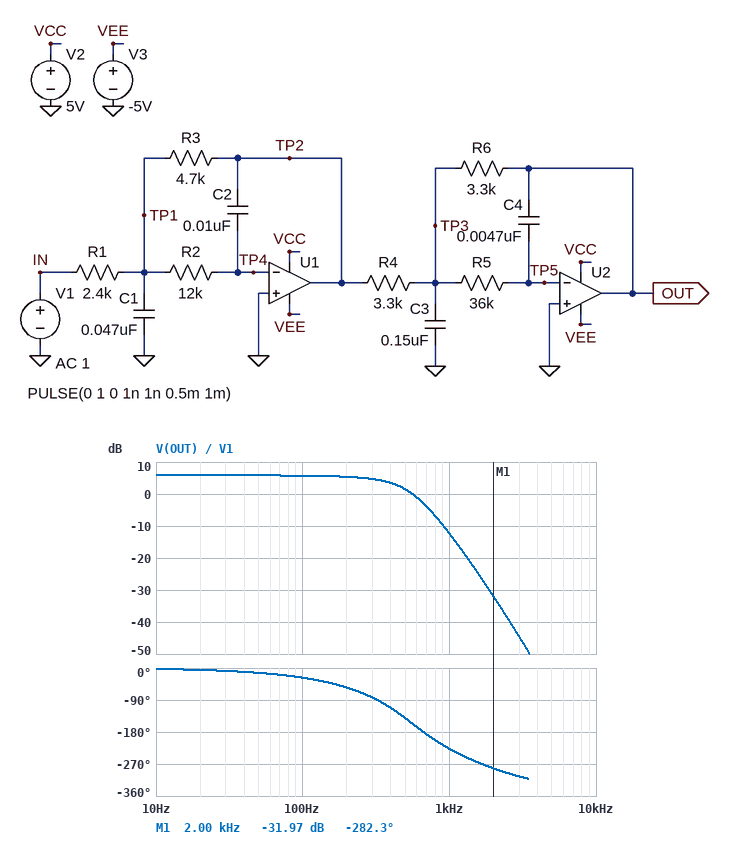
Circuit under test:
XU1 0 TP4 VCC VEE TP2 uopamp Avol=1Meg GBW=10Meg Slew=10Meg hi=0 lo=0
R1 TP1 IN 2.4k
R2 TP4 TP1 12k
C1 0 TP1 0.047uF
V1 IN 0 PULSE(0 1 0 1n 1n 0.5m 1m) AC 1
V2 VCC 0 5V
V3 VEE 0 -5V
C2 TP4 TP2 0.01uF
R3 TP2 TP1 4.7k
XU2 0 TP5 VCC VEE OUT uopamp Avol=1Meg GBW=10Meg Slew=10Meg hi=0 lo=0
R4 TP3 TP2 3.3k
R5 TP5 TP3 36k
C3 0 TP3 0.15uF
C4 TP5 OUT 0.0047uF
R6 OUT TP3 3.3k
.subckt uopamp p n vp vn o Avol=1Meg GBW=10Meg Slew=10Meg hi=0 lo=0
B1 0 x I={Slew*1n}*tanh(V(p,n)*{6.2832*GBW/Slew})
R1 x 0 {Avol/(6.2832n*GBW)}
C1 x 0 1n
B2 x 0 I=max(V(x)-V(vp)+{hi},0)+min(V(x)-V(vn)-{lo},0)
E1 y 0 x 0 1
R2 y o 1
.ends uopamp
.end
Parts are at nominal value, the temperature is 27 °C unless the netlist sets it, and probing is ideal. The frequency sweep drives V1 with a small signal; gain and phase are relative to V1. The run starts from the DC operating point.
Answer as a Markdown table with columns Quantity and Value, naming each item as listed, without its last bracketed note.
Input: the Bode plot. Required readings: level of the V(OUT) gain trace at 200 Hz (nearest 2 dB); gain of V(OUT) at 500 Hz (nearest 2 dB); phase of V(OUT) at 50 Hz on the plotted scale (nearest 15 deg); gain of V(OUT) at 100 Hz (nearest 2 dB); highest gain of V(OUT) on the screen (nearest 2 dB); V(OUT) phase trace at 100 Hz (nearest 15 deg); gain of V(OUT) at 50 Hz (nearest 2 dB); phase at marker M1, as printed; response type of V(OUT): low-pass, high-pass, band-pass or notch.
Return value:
| Quantity | Value |
|---|---|
| level of the V(OUT) gain trace at 200 Hz | 6 dB |
| gain of V(OUT) at 500 Hz | 2 dB |
| phase of V(OUT) at 50 Hz on the plotted scale | -15 deg |
| gain of V(OUT) at 100 Hz | 6 dB |
| highest gain of V(OUT) on the screen | 6 dB |
| V(OUT) phase trace at 100 Hz | -30 deg |
| gain of V(OUT) at 50 Hz | 6 dB |
| phase at marker M1, as printed | -282.3 deg |
| response type of V(OUT): low-pass, high-pass, band-pass or notch | low-pass |
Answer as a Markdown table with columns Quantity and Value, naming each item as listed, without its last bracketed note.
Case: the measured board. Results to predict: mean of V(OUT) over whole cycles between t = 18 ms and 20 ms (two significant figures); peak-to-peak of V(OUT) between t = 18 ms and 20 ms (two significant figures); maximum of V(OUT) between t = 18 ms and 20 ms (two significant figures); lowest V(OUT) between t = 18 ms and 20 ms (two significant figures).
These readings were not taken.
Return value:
| Quantity | Value |
|---|---|
| mean of V(OUT) over whole cycles between t = 18 ms and 20 ms | 980 mV |
| peak-to-peak of V(OUT) between t = 18 ms and 20 ms | 310 mV |
| maximum of V(OUT) between t = 18 ms and 20 ms | 1.1 V |
| lowest V(OUT) between t = 18 ms and 20 ms | 830 mV |
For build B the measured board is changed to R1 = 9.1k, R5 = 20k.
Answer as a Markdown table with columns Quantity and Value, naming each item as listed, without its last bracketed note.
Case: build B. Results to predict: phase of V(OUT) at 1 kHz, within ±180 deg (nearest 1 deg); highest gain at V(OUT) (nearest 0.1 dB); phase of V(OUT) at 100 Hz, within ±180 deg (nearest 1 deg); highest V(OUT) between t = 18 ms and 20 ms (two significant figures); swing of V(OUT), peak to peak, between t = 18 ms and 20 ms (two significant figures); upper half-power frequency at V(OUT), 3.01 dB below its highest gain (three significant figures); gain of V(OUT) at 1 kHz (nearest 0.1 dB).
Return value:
| Quantity | Value |
|---|---|
| phase of V(OUT) at 1 kHz, within ±180 deg | 145 deg |
| highest gain at V(OUT) | -4.5 dB |
| phase of V(OUT) at 100 Hz, within ±180 deg | -16 deg |
| highest V(OUT) between t = 18 ms and 20 ms | 410 mV |
| swing of V(OUT), peak to peak, between t = 18 ms and 20 ms | 300 mV |
| upper half-power frequency at V(OUT), 3.01 dB below its highest gain | 793 Hz |
| gain of V(OUT) at 1 kHz | -12.6 dB |
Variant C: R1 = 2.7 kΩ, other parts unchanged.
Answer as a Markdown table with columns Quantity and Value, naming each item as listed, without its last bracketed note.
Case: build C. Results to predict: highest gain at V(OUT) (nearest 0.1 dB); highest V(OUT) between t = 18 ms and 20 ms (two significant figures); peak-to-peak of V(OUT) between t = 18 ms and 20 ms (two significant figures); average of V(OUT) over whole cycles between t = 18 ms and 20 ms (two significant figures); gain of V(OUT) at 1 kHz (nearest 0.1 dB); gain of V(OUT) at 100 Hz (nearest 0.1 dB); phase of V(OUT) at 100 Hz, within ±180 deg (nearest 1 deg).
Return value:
| Quantity | Value |
|---|---|
| highest gain at V(OUT) | 4.8 dB |
| highest V(OUT) between t = 18 ms and 20 ms | 1.0 V |
| peak-to-peak of V(OUT) between t = 18 ms and 20 ms | 290 mV |
| average of V(OUT) over whole cycles between t = 18 ms and 20 ms | 870 mV |
| gain of V(OUT) at 1 kHz | -12.8 dB |
| gain of V(OUT) at 100 Hz | 4.7 dB |
| phase of V(OUT) at 100 Hz, within ±180 deg | -26 deg |
